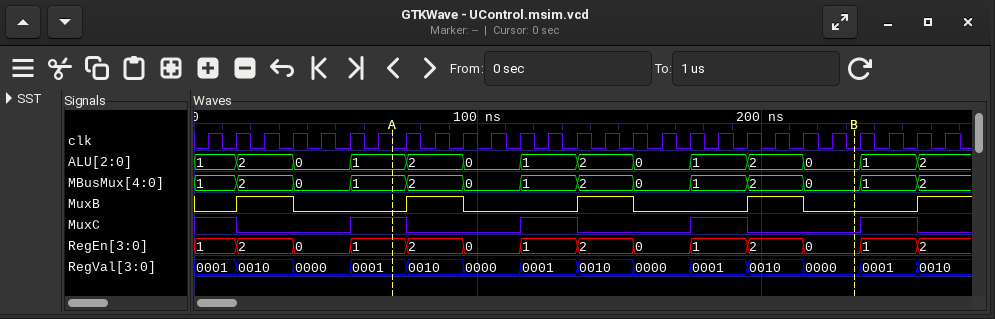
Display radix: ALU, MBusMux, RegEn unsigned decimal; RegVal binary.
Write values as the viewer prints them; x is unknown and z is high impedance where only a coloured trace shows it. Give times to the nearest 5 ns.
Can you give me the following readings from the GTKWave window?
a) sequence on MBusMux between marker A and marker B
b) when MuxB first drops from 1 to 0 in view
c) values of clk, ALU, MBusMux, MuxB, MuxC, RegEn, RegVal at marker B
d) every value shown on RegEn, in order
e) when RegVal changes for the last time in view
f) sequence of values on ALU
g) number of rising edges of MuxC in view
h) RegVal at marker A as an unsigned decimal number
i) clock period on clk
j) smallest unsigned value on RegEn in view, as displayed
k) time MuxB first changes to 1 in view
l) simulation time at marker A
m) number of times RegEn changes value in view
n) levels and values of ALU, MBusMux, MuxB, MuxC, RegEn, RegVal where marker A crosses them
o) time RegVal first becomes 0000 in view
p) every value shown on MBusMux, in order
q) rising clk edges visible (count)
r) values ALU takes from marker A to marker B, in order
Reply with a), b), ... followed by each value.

a) 1, 2, 0, 1, 2, 0, 1, 2, 0
b) 35 ns
c) clk=0, ALU=0, MBusMux=0, MuxB=0, MuxC=0, RegEn=0, RegVal=0000
d) 1, 2, 0, 1, 2, 0, 1, 2, 0, 1, 2, 0, 1, 2
e) 255 ns
f) 1, 2, 0, 1, 2, 0, 1, 2, 0, 1, 2, 0, 1, 2
g) 4
h) 1
i) 10 ns
j) 0
k) 15 ns
l) 70 ns
m) 13
n) ALU=1, MBusMux=1, MuxB=0, MuxC=1, RegEn=1, RegVal=0001
o) 35 ns
p) 1, 2, 0, 1, 2, 0, 1, 2, 0, 1, 2, 0, 1, 2
q) 27
r) 1, 2, 0, 1, 2, 0, 1, 2, 0
